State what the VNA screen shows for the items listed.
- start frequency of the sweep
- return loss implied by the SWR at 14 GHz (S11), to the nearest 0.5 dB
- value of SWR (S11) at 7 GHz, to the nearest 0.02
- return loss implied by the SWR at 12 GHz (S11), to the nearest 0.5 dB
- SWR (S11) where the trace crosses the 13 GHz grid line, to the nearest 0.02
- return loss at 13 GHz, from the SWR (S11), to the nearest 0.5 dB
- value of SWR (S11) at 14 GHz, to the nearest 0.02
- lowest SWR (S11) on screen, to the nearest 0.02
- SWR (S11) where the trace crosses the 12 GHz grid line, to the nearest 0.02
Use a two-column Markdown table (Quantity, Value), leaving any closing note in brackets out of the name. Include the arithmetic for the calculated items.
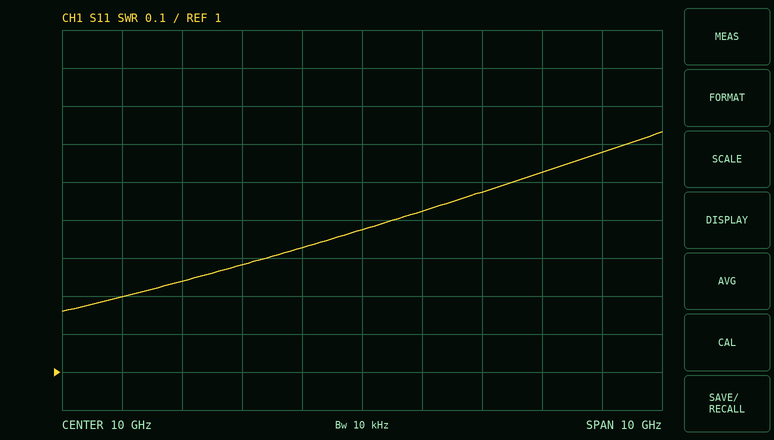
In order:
| Quantity | Value |
|---|---|
| start frequency of the sweep | 5 GHz |
| return loss implied by the SWR at 14 GHz (S11), to the nearest 0.5 dB | −20 log10((1.58 − 1)/(1.58 + 1)) ≈ 13.0 dB |
| value of SWR (S11) at 7 GHz, to the nearest 0.02 | 1.24 |
| return loss implied by the SWR at 12 GHz (S11), to the nearest 0.5 dB | −20 log10((1.48 − 1)/(1.48 + 1)) ≈ 14.3 dB, so 14.5 dB to the nearest 0.5 dB |
| SWR (S11) where the trace crosses the 13 GHz grid line, to the nearest 0.02 | 1.52 |
| return loss at 13 GHz, from the SWR (S11), to the nearest 0.5 dB | −20 log10((1.52 − 1)/(1.52 + 1)) ≈ 13.7 dB, so 13.5 dB to the nearest 0.5 dB |
| value of SWR (S11) at 14 GHz, to the nearest 0.02 | 1.58 |
| lowest SWR (S11) on screen, to the nearest 0.02 | 1.16 |
| SWR (S11) where the trace crosses the 12 GHz grid line, to the nearest 0.02 | 1.48 |
